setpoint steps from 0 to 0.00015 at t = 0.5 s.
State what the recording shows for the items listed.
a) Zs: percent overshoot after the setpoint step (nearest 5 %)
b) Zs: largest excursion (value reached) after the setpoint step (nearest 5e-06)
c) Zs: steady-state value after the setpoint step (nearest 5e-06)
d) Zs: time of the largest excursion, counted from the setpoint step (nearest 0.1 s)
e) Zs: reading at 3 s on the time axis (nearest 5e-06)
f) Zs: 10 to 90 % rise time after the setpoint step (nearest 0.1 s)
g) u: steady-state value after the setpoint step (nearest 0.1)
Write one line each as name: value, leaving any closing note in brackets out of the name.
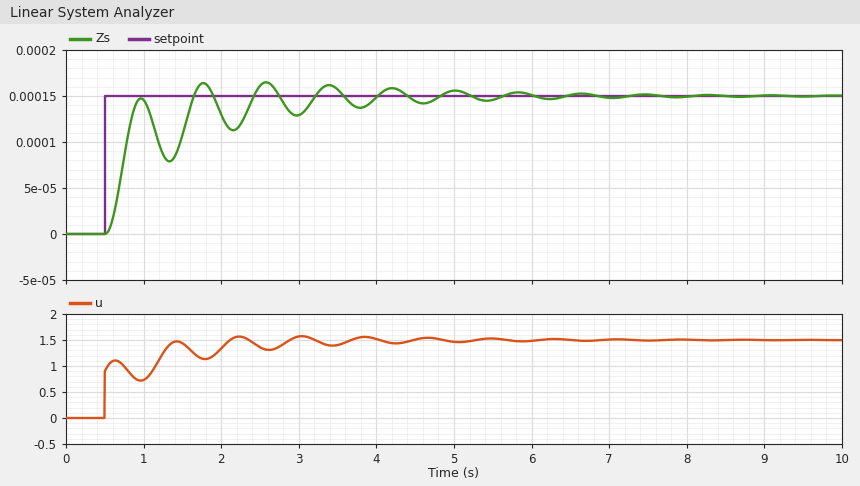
Zs: percent overshoot after the setpoint step: 10 %
Zs: largest excursion (value reached) after the setpoint step: 0.000165
Zs: steady-state value after the setpoint step: 0.000150
Zs: time of the largest excursion, counted from the setpoint step: 2.1 s
Zs: reading at 3 s on the time axis: 0.000130
Zs: 10 to 90 % rise time after the setpoint step: 0.3 s
u: steady-state value after the setpoint step: 1.5
